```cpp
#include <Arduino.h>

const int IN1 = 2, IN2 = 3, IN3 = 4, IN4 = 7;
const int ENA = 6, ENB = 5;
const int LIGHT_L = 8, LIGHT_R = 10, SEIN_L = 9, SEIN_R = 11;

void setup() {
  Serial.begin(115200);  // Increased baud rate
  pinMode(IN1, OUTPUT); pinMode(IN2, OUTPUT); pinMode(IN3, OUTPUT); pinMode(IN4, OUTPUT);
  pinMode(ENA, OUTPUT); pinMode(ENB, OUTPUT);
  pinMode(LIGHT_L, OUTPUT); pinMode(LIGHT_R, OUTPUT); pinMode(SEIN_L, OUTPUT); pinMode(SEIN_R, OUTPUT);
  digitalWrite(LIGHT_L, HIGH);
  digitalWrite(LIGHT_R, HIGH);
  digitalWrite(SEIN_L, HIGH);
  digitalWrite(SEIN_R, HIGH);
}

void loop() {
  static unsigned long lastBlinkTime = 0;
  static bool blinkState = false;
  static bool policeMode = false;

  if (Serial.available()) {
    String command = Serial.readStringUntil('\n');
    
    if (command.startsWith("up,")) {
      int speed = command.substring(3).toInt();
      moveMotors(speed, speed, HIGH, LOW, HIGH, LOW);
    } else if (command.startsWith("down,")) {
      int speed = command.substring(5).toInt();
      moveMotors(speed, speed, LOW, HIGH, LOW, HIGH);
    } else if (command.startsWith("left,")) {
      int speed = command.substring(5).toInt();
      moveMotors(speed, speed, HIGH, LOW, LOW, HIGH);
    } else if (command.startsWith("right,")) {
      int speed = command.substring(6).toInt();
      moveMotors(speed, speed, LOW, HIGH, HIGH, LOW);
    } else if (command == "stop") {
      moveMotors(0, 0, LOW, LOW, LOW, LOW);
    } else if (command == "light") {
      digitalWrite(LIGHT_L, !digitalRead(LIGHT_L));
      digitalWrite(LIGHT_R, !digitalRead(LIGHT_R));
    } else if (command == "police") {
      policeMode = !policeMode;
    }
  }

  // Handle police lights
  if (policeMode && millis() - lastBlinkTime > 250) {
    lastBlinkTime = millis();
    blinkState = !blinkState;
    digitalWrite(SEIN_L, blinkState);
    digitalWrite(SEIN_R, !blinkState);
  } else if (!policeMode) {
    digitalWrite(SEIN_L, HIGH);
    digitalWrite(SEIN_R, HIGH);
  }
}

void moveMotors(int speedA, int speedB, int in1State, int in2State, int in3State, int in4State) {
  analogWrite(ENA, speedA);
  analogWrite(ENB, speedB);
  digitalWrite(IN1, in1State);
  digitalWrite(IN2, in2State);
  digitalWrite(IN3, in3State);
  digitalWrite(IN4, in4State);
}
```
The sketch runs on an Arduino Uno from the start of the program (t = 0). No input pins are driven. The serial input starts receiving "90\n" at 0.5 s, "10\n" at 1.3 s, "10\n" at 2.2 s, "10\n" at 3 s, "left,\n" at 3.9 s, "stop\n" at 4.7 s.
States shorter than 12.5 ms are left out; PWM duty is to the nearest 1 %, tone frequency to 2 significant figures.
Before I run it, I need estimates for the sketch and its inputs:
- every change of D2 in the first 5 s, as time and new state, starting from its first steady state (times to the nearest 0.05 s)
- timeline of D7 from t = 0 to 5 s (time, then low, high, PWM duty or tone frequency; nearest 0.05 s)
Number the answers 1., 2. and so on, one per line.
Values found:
1. 0 s low; 3.9 s high; 4.7 s low
2. 0 s low; 3.9 s high; 4.7 s low
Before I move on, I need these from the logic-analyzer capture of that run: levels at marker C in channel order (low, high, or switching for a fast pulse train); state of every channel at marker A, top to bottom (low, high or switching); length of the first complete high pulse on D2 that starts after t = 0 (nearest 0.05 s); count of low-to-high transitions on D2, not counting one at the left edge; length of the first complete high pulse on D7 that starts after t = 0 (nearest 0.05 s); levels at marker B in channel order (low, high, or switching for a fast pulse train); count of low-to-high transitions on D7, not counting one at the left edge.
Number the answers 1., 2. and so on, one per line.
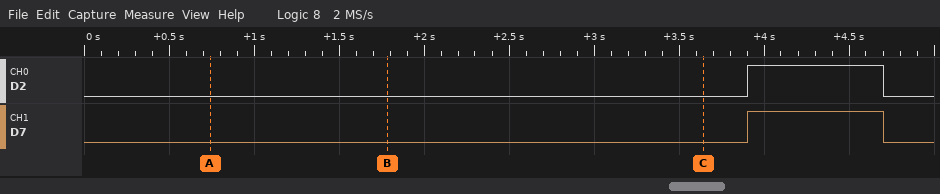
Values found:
1. D2 low, D7 low
2. D2 low, D7 low
3. 0.80 s
4. 1
5. 0.80 s
6. D2 low, D7 low
7. 1
